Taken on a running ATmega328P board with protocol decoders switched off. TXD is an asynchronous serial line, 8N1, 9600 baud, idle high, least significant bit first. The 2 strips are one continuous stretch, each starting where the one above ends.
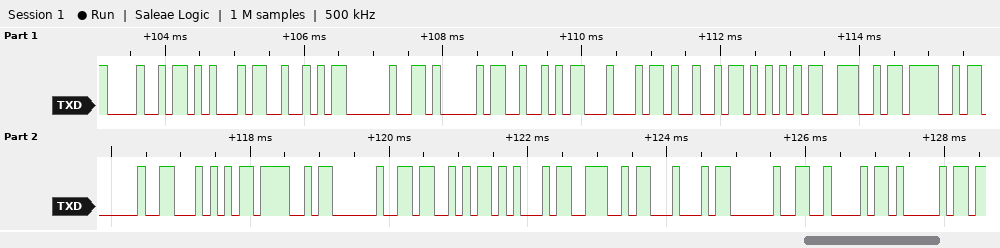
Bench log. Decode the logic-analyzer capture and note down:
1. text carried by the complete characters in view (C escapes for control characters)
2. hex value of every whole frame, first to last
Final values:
"HER ARDIUNO TO SEND BA"
0x48 0x45 0x52 0x20 0x41 0x52 0x44 0x49 0x55 0x4E 0x4F 0x20 0x54 0x4F 0x20 0x53 0x45 0x4E 0x44 0x20 0x42 0x41
